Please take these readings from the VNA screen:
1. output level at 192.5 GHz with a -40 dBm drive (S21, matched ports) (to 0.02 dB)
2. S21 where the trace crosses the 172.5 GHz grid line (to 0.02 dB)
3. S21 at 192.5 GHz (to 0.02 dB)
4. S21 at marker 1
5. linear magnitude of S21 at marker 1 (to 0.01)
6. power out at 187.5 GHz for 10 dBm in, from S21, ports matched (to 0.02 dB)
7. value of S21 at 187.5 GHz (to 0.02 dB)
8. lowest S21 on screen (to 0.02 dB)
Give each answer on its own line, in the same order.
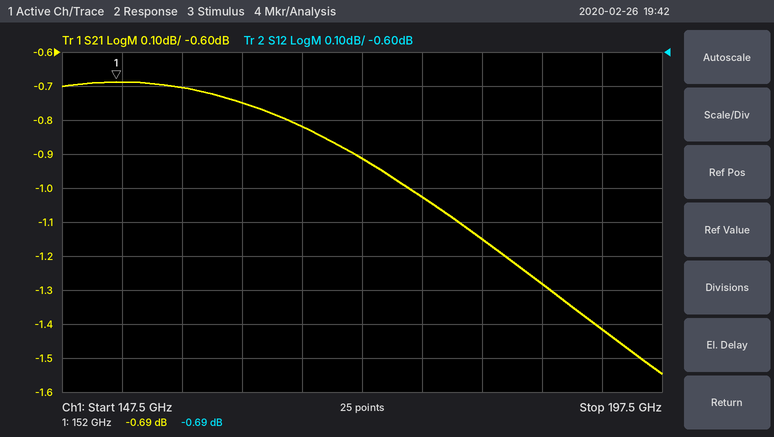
-41.42 dBm
-0.92 dB
-1.42 dB
-0.69 dB
0.92
8.72 dBm
-1.28 dB
-1.54 dB
